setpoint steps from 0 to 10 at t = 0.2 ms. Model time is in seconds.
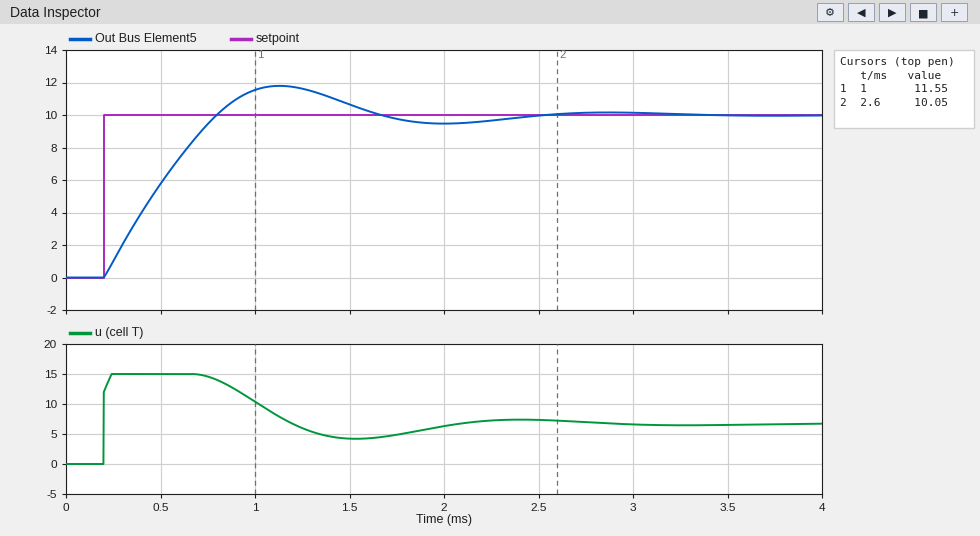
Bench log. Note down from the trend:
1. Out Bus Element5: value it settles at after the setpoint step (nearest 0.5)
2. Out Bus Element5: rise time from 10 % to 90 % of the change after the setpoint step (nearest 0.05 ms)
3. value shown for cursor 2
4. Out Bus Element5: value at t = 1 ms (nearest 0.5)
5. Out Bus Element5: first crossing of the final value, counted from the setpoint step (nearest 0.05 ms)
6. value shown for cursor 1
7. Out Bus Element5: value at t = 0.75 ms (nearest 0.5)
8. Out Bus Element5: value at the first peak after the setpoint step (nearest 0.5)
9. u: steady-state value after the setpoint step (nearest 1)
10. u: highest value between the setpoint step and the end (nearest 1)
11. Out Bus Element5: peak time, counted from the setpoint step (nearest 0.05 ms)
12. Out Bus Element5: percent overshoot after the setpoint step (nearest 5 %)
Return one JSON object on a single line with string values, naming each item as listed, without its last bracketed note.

{"Out Bus Element5: value it settles at after the setpoint step": "10.0", "Out Bus Element5: rise time from 10 % to 90 % of the change after the setpoint step": "0.45 ms", "value shown for cursor 2": "10.05", "Out Bus Element5: value at t = 1 ms": "11.5", "Out Bus Element5: first crossing of the final value, counted from the setpoint step": "0.60 ms", "value shown for cursor 1": "11.55", "Out Bus Element5: value at t = 0.75 ms": "9.5", "Out Bus Element5: value at the first peak after the setpoint step": "12.0", "u: steady-state value after the setpoint step": "7", "u: highest value between the setpoint step and the end": "15", "Out Bus Element5: peak time, counted from the setpoint step": "0.95 ms", "Out Bus Element5: percent overshoot after the setpoint step": "20 %"}
